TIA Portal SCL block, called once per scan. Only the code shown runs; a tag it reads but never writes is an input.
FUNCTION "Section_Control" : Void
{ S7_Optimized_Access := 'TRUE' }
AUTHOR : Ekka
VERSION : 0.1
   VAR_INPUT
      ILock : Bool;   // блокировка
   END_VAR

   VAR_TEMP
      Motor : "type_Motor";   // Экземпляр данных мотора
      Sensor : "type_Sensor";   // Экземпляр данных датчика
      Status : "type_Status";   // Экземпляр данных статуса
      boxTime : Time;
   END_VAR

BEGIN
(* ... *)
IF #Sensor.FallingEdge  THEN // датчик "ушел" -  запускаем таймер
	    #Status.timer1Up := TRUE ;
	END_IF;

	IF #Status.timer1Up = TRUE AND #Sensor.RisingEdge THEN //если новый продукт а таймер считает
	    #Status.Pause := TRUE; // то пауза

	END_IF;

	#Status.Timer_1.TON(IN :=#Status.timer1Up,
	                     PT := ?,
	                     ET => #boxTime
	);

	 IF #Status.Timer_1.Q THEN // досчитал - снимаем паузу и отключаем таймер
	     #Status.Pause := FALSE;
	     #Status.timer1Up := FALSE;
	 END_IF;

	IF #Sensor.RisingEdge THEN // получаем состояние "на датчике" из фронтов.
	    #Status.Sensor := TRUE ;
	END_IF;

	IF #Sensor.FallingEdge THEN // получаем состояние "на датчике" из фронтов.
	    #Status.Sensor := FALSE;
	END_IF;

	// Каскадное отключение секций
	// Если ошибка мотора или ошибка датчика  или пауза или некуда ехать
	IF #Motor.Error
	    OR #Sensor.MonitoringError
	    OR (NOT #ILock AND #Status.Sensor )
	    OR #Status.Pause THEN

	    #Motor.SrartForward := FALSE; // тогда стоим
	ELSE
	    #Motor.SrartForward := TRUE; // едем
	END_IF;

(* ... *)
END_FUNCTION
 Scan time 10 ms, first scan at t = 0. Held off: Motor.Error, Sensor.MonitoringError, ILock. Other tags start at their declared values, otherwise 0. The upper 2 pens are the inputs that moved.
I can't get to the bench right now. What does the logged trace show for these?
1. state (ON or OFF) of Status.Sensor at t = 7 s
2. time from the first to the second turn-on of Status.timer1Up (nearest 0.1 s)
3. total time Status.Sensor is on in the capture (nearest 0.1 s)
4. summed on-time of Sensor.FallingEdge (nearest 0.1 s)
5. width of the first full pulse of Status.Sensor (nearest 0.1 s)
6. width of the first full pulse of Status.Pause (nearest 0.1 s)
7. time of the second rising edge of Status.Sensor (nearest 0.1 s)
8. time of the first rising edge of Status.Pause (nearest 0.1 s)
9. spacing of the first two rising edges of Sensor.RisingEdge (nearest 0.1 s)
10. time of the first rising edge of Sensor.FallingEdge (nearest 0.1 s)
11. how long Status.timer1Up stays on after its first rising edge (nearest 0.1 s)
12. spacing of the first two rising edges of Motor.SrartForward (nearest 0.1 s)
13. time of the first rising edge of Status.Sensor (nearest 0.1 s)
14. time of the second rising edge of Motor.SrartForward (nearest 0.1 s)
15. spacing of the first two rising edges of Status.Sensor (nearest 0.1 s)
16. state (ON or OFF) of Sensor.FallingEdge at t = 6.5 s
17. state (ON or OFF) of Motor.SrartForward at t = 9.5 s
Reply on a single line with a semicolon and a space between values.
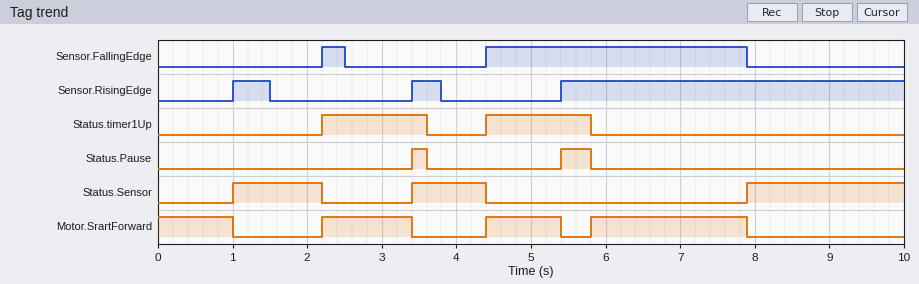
OFF; 2.2 s; 4.3 s; 3.8 s; 1.2 s; 0.2 s; 3.4 s; 3.4 s; 2.4 s; 2.2 s; 1.4 s; 2.2 s; 1.0 s; 4.4 s; 2.4 s; ON; OFF
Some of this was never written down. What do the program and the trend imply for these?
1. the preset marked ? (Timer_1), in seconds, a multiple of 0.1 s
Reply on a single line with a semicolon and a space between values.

1.4 s
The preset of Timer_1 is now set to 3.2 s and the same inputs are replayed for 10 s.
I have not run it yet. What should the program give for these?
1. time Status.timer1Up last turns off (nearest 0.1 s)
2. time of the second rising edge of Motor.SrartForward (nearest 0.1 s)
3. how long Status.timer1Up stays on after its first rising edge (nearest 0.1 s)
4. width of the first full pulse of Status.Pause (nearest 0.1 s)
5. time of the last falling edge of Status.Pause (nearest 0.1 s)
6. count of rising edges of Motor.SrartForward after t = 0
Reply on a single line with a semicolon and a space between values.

5.4 s; 5.4 s; 3.2 s; 2.0 s; 5.4 s; 2
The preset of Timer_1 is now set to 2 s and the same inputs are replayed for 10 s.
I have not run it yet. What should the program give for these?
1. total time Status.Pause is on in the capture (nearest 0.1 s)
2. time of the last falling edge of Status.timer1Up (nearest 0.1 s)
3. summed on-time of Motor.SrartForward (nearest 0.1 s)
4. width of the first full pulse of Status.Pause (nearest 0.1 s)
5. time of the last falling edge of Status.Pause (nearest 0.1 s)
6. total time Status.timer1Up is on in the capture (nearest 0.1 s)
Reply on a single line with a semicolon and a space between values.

1.8 s; 6.4 s; 4.7 s; 0.8 s; 6.4 s; 4.0 s
